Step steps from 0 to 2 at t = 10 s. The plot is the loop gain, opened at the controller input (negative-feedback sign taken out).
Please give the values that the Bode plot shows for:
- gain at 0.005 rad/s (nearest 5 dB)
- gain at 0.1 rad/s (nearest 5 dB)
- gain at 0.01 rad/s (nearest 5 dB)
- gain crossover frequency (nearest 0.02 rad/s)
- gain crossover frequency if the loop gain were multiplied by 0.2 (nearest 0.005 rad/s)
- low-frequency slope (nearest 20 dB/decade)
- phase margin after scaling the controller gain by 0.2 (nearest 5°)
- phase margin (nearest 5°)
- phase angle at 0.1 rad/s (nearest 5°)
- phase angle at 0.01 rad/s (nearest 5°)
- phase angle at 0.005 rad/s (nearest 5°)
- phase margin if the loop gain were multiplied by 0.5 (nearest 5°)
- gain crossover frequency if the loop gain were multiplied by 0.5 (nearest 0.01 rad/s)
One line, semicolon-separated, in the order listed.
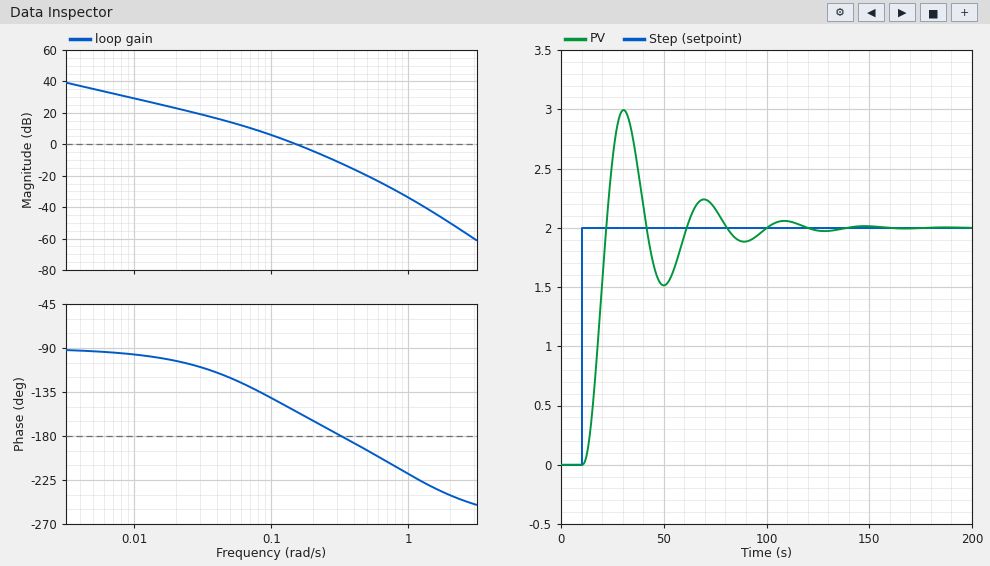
35 dB; 5 dB; 30 dB; 0.16 rad/s; 0.050 rad/s; -20 dB/decade; 60°; 25°; -140°; -95°; -95°; 40°; 0.10 rad/s
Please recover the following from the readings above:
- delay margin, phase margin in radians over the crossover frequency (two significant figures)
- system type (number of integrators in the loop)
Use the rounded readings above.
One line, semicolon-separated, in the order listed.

2.7 s; 1
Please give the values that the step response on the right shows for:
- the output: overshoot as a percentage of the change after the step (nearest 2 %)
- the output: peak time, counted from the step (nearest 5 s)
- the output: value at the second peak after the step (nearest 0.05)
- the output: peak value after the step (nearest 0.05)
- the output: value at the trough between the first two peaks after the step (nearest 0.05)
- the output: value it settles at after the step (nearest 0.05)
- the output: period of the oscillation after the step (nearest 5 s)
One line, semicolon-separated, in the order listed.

50 %; 20 s; 2.25; 3.00; 1.50; 2.00; 40 s
